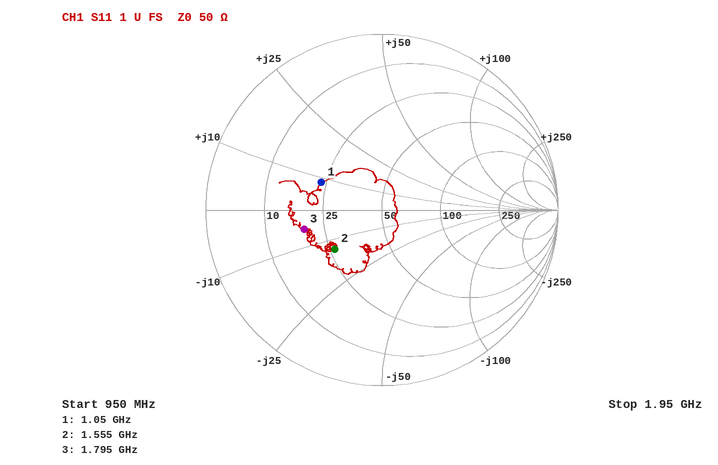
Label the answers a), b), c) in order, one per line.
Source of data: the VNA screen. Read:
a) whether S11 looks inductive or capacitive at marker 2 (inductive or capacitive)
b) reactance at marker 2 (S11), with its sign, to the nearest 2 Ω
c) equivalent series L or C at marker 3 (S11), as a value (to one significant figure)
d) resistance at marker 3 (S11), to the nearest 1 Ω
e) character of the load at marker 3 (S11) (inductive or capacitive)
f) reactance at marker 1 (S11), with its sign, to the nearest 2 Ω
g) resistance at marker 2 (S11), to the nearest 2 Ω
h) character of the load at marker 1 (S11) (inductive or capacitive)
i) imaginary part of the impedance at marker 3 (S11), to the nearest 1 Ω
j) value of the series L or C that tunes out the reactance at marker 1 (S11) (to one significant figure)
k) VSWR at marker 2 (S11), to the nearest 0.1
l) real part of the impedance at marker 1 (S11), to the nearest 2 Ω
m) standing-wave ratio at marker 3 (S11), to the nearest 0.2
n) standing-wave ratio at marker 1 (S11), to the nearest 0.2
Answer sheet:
a) capacitive
b) -14 Ω
c) 20 pF
d) 19 Ω
e) capacitive
f) +8 Ω
g) 26 Ω
h) inductive
i) -5 Ω
j) 20 pF
k) 2.1
l) 24 Ω
m) 2.6
n) 2.2
